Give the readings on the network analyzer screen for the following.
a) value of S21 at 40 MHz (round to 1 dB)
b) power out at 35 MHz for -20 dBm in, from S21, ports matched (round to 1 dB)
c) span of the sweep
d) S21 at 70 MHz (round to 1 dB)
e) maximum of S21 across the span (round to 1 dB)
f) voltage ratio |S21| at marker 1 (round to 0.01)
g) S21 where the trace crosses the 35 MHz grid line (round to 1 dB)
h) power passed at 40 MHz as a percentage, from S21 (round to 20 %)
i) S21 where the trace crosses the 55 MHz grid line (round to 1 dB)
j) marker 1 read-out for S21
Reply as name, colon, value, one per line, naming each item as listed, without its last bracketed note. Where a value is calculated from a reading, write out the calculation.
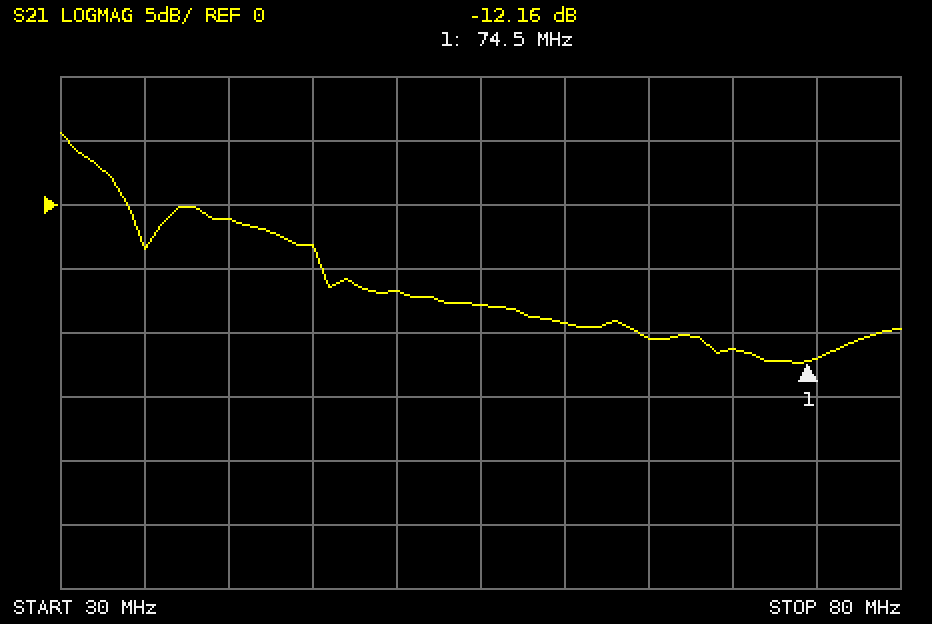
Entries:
value of S21 at 40 MHz: -1 dB
power out at 35 MHz for -20 dBm in, from S21, ports matched: -20 dBm + (-3 dB) = -23 dBm
span of the sweep: 50 MHz
S21 at 70 MHz: -11 dB
maximum of S21 across the span: 6 dB
voltage ratio |S21| at marker 1: 10^(-12.16/20) ≈ 0.25
S21 where the trace crosses the 35 MHz grid line: -3 dB
power passed at 40 MHz as a percentage, from S21: 10^(-1/10) ≈ 79.4 %, so 80 % to the nearest 20 %
S21 where the trace crosses the 55 MHz grid line: -8 dB
marker 1 read-out for S21: -12.16 dB
